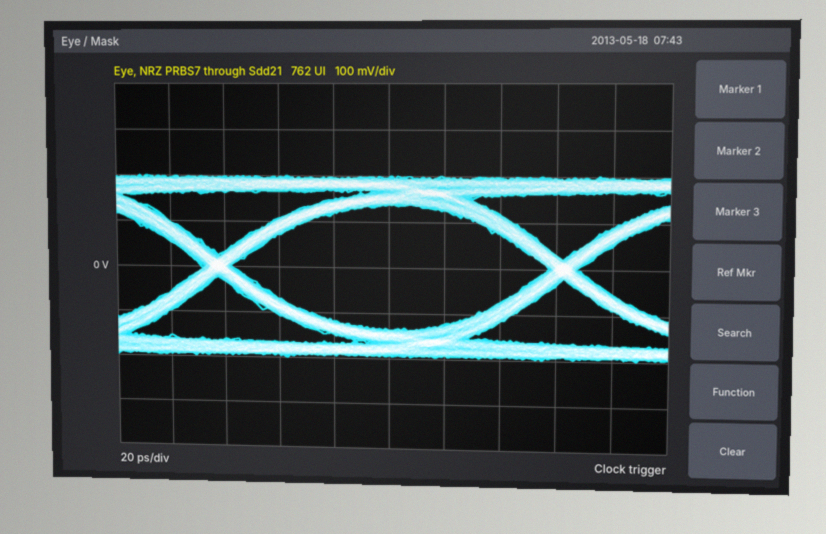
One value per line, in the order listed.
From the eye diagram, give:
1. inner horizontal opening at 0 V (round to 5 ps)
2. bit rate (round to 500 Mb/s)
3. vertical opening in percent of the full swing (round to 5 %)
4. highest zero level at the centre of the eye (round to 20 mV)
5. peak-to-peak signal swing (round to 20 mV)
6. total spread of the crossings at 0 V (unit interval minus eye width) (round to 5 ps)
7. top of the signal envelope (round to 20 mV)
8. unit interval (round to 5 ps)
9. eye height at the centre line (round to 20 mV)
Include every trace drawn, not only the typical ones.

115 ps
8.0 Gb/s
70 %
-140 mV
400 mV
10 ps
200 mV
125 ps
280 mV
